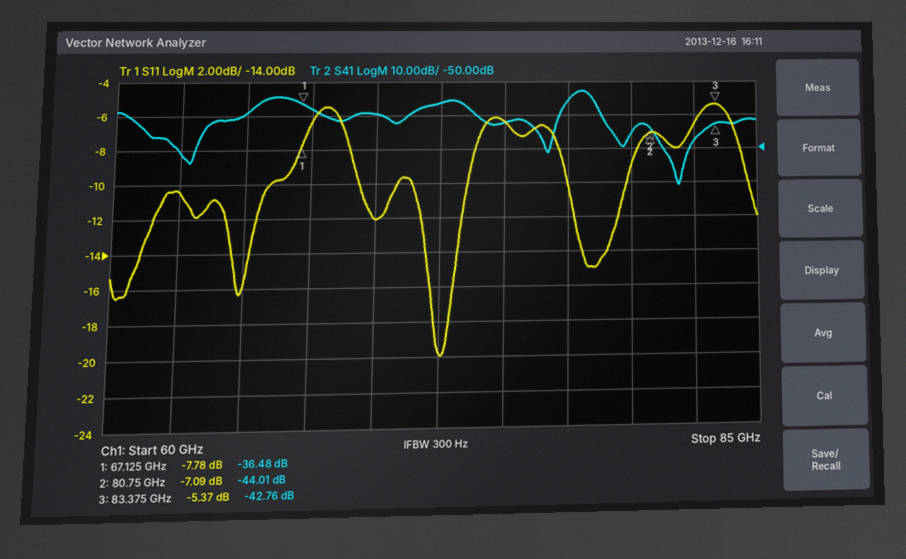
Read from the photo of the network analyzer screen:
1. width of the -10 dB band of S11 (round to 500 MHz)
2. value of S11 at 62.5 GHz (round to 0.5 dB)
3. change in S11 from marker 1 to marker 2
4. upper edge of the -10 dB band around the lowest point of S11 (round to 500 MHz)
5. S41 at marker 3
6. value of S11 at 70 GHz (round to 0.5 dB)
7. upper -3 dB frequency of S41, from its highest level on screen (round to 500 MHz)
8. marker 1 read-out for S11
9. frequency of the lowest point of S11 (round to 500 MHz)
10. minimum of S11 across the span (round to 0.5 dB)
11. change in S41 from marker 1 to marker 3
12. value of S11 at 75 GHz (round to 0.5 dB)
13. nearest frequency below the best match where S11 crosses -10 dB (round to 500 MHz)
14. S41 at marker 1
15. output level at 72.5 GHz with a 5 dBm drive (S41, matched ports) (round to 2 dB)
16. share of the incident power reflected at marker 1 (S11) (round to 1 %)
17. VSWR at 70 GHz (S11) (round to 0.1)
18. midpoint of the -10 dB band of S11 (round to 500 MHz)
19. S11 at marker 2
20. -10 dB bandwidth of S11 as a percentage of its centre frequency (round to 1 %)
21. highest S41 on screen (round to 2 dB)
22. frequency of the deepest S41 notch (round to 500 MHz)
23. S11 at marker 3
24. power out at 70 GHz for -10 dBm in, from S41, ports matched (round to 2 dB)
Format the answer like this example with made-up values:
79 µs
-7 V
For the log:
2.0 GHz
-10.5 dB
0.69 dB
73.5 GHz
-42.76 dB
-12.0 dB
78.5 GHz
-7.78 dB
72.5 GHz
-20.0 dB
-6.28 dB
-6.5 dB
71.5 GHz
-36.48 dB
-32 dBm
17 %
1.7
72.5 GHz
-7.09 dB
3 %
-32 dB
82.0 GHz
-5.37 dB
-50 dBm
